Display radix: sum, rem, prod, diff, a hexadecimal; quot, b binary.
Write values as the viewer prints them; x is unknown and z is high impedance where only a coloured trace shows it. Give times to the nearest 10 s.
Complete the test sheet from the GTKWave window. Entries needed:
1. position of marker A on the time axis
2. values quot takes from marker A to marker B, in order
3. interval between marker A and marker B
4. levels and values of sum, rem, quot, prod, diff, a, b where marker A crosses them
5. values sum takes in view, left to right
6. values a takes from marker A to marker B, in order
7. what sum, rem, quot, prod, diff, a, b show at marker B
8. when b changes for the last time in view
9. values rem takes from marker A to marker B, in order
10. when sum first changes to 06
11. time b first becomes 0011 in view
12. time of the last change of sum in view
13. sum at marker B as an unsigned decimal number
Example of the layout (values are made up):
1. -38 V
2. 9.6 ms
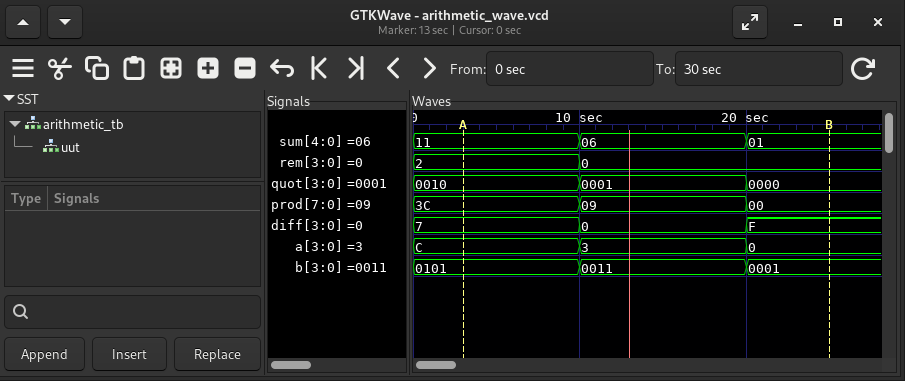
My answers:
1. 0 s
2. 0010, 0001, 0000
3. 20 s
4. sum=11, rem=2, quot=0010, prod=3C, diff=7, a=C, b=0101
5. 11, 06, 01
6. C, 3, 0
7. sum=01, rem=0, quot=0000, prod=00, diff=F, a=0, b=0001
8. 20 s
9. 2, 0
10. 10 s
11. 10 s
12. 20 s
13. 1
